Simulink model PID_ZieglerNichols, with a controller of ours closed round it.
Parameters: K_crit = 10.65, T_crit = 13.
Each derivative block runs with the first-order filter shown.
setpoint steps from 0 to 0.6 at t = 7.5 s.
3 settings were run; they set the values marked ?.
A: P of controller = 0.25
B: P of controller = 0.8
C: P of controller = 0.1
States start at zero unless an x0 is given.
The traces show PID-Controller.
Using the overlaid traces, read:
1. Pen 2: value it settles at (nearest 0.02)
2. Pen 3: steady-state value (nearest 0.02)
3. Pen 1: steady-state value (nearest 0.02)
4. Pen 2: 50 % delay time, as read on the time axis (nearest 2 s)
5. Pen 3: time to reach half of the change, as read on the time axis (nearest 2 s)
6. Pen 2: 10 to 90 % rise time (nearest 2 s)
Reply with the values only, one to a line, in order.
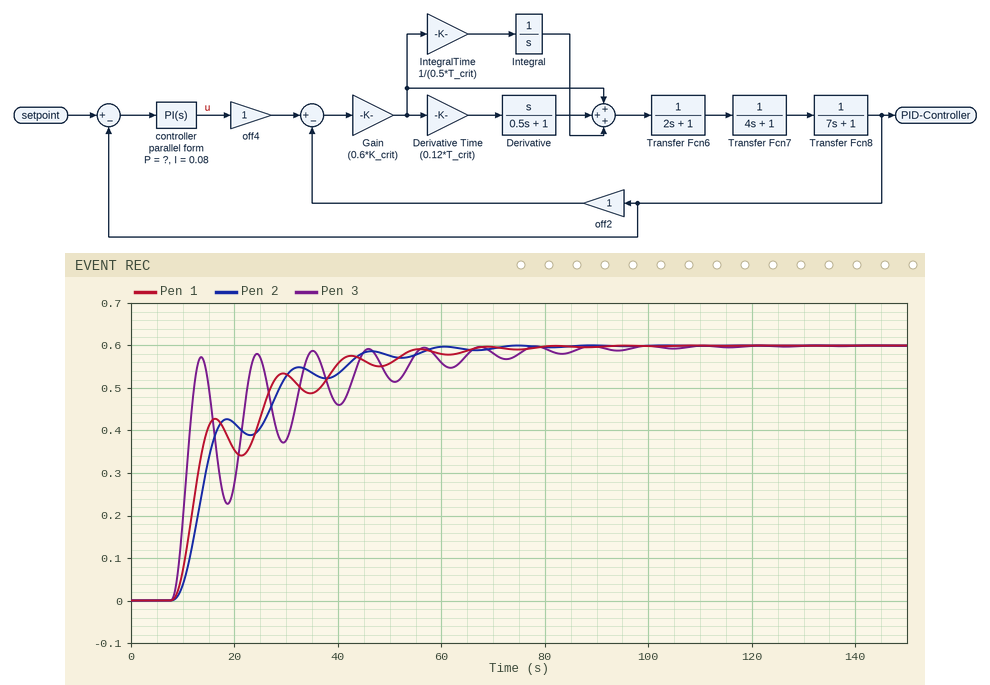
0.60
0.60
0.60
14 s
10 s
20 s
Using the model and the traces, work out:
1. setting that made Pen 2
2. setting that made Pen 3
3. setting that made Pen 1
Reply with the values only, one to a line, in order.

C
B
A
